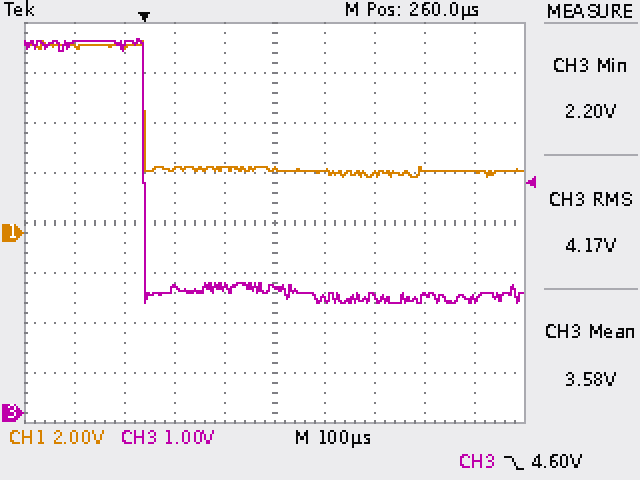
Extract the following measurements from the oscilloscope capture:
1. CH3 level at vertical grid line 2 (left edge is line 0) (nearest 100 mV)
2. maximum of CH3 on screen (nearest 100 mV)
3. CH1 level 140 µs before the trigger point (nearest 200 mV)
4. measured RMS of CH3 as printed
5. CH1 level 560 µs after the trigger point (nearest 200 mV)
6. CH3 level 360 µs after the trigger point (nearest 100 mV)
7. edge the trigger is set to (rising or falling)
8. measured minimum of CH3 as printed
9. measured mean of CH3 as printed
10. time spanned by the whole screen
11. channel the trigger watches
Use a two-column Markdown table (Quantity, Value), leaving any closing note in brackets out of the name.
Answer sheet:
| Quantity | Value |
|---|---|
| CH3 level at vertical grid line 2 (left edge is line 0) | 7.3 V |
| maximum of CH3 on screen | 7.5 V |
| CH1 level 140 µs before the trigger point | 7.4 V |
| measured RMS of CH3 as printed | 4.17 V |
| CH1 level 560 µs after the trigger point | 2.6 V |
| CH3 level 360 µs after the trigger point | 2.3 V |
| edge the trigger is set to | falling |
| measured minimum of CH3 as printed | 2.20 V |
| measured mean of CH3 as printed | 3.58 V |
| time spanned by the whole screen | 1 ms |
| channel the trigger watches | CH3 |
